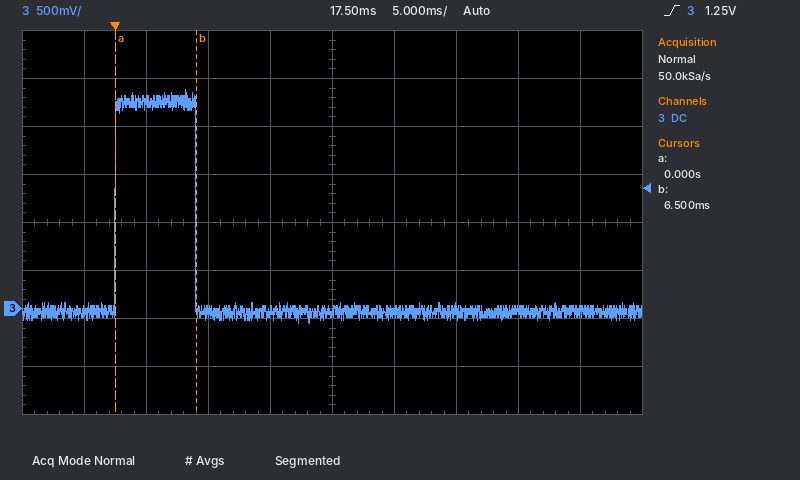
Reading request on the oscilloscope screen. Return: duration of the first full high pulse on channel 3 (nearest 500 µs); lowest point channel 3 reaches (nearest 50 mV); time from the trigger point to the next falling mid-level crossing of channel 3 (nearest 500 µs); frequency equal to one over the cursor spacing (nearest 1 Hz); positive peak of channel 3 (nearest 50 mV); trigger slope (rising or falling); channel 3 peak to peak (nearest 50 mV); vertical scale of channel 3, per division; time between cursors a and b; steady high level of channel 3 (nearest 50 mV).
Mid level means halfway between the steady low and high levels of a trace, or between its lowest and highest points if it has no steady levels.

6.5 ms
-150 mV
6.5 ms
154 Hz
2.30 V
rising
2.45 V
500 mV
6.5 ms
2.15 V
